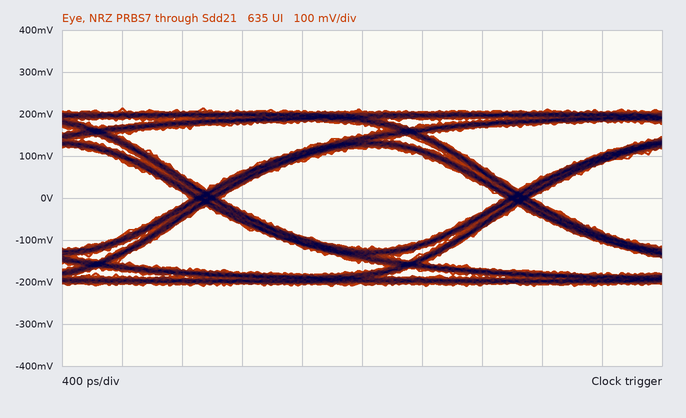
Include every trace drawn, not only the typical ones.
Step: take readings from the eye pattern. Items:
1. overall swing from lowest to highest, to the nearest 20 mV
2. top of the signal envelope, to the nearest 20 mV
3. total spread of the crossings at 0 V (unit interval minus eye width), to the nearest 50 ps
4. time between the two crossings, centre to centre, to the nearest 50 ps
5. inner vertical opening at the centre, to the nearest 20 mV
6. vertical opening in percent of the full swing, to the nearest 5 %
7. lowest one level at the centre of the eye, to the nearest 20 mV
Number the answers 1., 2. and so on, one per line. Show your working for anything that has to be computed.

1. 420 mV
2. 220 mV
3. 200 ps
4. 2.10 ns
5. 240 mV
6. 240 mV / 420 mV ≈ 57.1 %, so 55 % to the nearest 5 %
7. 120 mV
